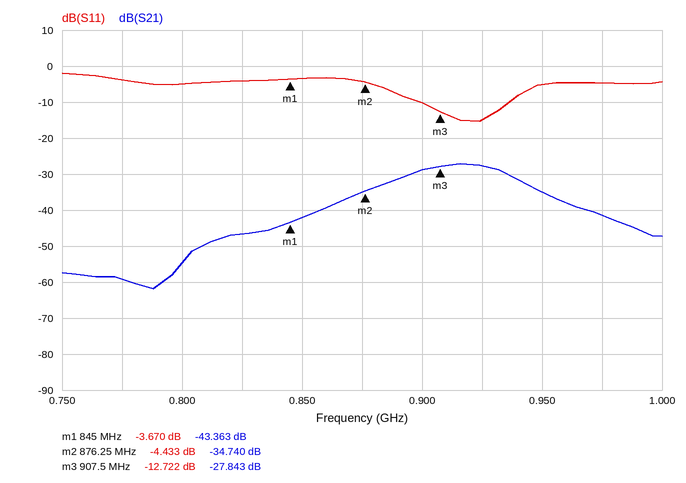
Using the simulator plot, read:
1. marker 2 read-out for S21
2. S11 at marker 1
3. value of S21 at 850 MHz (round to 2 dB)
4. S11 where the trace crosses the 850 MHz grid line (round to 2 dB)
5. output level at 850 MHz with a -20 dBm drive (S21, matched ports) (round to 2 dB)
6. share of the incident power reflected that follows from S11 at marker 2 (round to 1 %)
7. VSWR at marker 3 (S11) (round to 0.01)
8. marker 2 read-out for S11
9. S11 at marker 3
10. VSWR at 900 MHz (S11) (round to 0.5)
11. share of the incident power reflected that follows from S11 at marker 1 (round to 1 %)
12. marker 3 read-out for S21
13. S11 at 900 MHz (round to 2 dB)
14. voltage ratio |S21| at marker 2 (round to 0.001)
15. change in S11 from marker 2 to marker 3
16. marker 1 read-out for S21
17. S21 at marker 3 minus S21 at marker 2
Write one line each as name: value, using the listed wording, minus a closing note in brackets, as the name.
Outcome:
marker 2 read-out for S21: -34.740 dB
S11 at marker 1: -3.670 dB
value of S21 at 850 MHz: -42 dB
S11 where the trace crosses the 850 MHz grid line: -4 dB
output level at 850 MHz with a -20 dBm drive (S21, matched ports): -62 dBm
share of the incident power reflected that follows from S11 at marker 2: 36 %
VSWR at marker 3 (S11): 1.60
marker 2 read-out for S11: -4.433 dB
S11 at marker 3: -12.722 dB
VSWR at 900 MHz (S11): 2.0
share of the incident power reflected that follows from S11 at marker 1: 43 %
marker 3 read-out for S21: -27.843 dB
S11 at 900 MHz: -10 dB
voltage ratio |S21| at marker 2: 0.018
change in S11 from marker 2 to marker 3: -8.289 dB
marker 1 read-out for S21: -43.363 dB
S21 at marker 3 minus S21 at marker 2: 6.897 dB
